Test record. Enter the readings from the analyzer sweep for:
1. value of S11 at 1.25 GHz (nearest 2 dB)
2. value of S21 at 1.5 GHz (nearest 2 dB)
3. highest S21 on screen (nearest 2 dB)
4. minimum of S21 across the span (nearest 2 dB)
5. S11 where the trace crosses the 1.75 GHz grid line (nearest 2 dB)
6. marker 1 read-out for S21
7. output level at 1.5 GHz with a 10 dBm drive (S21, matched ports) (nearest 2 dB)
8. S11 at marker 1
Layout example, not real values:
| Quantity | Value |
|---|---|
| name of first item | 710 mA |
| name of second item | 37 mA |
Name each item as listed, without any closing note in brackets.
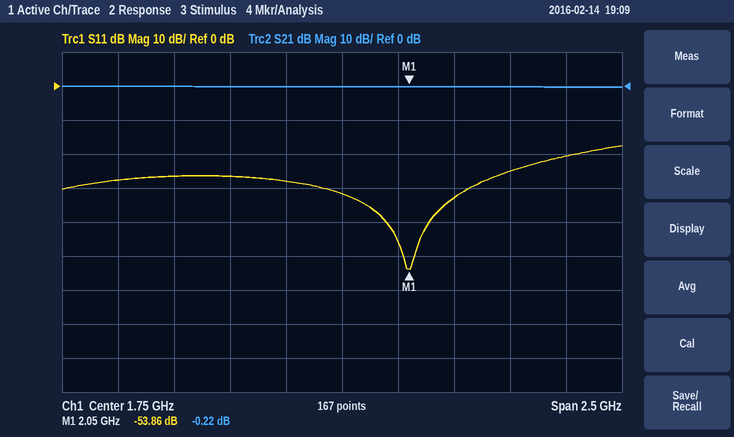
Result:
| Quantity | Value |
|---|---|
| value of S11 at 1.25 GHz | -26 dB |
| value of S21 at 1.5 GHz | 0 dB |
| highest S21 on screen | 0 dB |
| minimum of S21 across the span | 0 dB |
| S11 where the trace crosses the 1.75 GHz grid line | -32 dB |
| marker 1 read-out for S21 | -0.22 dB |
| output level at 1.5 GHz with a 10 dBm drive (S21, matched ports) | 10 dBm |
| S11 at marker 1 | -53.86 dB |
